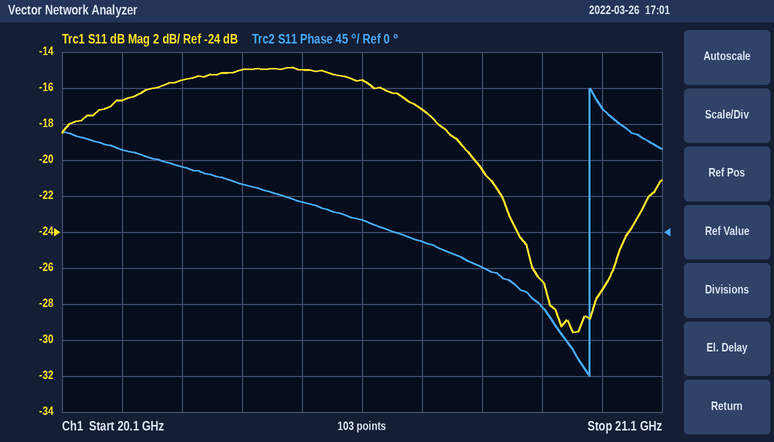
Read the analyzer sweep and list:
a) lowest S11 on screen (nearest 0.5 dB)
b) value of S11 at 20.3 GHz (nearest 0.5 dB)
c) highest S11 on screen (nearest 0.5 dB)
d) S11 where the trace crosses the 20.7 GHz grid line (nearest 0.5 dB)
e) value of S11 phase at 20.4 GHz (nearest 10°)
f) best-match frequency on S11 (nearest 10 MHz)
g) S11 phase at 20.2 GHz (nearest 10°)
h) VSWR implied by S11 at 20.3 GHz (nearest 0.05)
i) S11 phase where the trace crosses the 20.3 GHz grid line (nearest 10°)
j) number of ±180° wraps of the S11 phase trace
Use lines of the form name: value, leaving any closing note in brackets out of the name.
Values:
lowest S11 on screen: -29.5 dB
value of S11 at 20.3 GHz: -15.5 dB
highest S11 on screen: -15.0 dB
S11 where the trace crosses the 20.7 GHz grid line: -17.0 dB
value of S11 phase at 20.4 GHz: 60°
best-match frequency on S11: 20.95 GHz
S11 phase at 20.2 GHz: 100°
VSWR implied by S11 at 20.3 GHz: 1.40
S11 phase where the trace crosses the 20.3 GHz grid line: 80°
number of ±180° wraps of the S11 phase trace: 1
